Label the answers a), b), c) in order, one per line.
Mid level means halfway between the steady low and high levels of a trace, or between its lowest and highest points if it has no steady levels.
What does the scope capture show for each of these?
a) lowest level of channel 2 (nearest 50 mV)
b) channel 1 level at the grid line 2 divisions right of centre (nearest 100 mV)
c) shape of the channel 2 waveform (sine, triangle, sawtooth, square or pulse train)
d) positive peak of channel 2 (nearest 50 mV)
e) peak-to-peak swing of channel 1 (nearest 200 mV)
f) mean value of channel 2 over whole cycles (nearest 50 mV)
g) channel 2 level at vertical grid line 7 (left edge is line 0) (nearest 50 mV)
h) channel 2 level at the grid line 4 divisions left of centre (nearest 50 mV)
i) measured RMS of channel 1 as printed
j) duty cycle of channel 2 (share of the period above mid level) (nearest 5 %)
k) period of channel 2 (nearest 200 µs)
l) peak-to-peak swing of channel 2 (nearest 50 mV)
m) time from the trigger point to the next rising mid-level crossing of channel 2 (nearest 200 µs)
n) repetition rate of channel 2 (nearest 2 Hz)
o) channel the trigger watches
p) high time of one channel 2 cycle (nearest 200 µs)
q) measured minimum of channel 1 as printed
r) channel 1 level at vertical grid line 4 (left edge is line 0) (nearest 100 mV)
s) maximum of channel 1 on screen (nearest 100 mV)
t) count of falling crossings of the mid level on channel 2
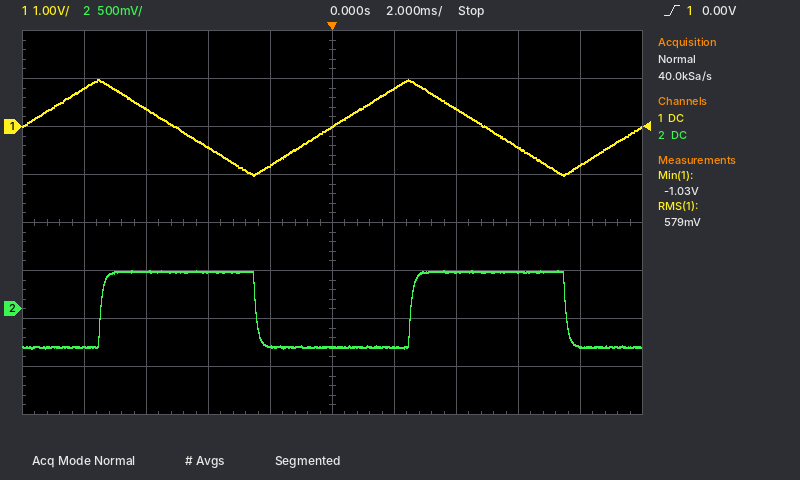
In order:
a) -400 mV
b) 400 mV
c) square
d) 400 mV
e) 2.0 V
f) 0 mV
g) 400 mV
h) -400 mV
i) 579 mV
j) 50 %
k) 10.0 ms
l) 800 mV
m) 2.6 ms
n) 100 Hz
o) channel 1
p) 5.0 ms
q) -1.03 V
r) -800 mV
s) 1.0 V
t) 2
